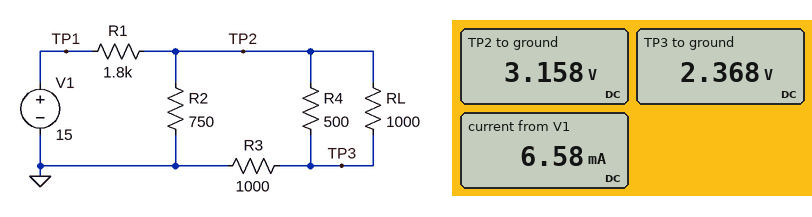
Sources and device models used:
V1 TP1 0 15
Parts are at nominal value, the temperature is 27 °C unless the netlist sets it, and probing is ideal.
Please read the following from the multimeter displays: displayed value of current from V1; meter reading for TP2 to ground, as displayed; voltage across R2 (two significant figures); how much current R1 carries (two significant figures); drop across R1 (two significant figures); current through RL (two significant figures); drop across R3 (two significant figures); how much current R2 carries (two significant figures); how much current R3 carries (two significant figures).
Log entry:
6.58 mA
3.158 V
3.2 V
6.6 mA
12 V
790 µA
2.4 V
4.2 mA
2.4 mA
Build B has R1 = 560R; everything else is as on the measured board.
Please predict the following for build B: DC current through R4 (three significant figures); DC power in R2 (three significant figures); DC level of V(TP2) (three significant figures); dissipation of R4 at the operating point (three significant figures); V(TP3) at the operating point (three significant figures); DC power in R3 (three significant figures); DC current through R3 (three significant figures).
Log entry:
3.46 mA
63.9 mW
6.92 V
5.99 mW
5.19 V
27.0 mW
5.19 mA
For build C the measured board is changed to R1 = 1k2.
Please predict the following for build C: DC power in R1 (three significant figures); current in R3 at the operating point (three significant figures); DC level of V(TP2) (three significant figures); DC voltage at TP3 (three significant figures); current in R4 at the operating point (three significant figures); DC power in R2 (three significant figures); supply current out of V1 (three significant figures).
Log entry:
95.7 mW
3.21 mA
4.29 V
3.21 V
2.14 mA
24.5 mW
8.93 mA
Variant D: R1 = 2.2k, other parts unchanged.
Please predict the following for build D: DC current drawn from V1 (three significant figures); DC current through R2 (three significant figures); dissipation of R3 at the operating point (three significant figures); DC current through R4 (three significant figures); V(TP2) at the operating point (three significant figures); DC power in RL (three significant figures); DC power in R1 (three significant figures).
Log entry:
5.60 mA
3.58 mA
4.06 mW
1.34 mA
2.69 V
451 µW
68.9 mW
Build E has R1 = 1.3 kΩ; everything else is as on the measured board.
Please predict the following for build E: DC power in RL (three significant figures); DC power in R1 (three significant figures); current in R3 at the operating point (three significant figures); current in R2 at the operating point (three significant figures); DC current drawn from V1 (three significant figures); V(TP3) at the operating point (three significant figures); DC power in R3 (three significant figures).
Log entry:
1.02 mW
92.3 mW
3.03 mA
5.39 mA
8.43 mA
3.03 V
9.20 mW
